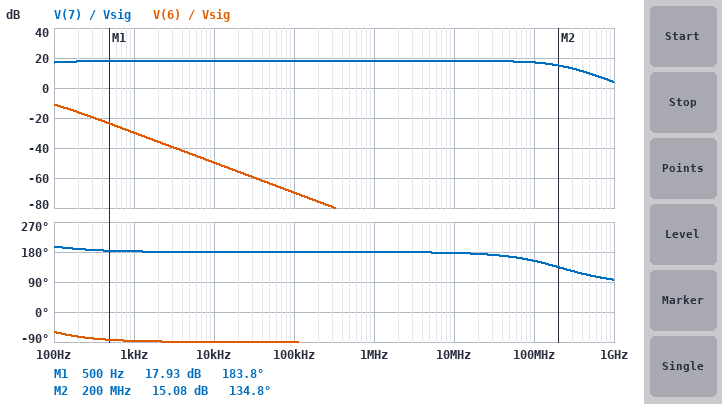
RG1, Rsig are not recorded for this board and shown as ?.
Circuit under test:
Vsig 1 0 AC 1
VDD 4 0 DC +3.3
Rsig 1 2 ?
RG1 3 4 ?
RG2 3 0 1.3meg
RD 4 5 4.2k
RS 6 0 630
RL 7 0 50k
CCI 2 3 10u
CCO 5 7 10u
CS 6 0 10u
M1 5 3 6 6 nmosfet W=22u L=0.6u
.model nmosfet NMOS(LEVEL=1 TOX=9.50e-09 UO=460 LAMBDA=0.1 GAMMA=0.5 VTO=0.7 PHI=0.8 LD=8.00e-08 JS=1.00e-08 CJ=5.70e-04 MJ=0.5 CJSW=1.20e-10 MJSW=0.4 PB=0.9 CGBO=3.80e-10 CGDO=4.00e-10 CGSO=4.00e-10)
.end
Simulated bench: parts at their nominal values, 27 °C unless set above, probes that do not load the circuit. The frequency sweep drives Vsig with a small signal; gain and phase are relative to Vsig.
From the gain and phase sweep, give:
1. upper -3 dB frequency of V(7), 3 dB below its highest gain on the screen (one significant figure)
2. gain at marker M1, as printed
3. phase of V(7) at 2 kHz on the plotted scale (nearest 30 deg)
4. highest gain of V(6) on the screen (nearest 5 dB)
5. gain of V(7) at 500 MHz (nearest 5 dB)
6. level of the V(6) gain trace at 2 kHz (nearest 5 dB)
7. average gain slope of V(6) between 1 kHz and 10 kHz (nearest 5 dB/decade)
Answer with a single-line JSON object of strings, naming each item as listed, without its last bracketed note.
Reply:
{"upper -3 dB frequency of V(7), 3 dB below its highest gain on the screen": "200 MHz", "gain at marker M1, as printed": "17.93 dB", "phase of V(7) at 2 kHz on the plotted scale": "180 deg", "highest gain of V(6) on the screen": "-10 dB", "gain of V(7) at 500 MHz": "10 dB", "level of the V(6) gain trace at 2 kHz": "-35 dB", "average gain slope of V(6) between 1 kHz and 10 kHz": "-20 dB/decade"}
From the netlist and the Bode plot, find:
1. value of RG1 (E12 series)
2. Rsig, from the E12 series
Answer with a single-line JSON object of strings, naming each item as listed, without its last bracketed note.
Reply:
{"value of RG1": "2.7 MΩ", "Rsig, from the E12 series": "6.8 kΩ"}
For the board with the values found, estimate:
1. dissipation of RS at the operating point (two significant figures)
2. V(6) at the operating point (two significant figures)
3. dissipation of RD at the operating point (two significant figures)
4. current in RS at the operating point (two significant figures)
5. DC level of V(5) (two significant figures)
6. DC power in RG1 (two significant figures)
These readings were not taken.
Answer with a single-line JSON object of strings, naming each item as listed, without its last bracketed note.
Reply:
{"dissipation of RS at the operating point": "37 µW", "V(6) at the operating point": "150 mV", "dissipation of RD at the operating point": "250 µW", "current in RS at the operating point": "240 µA", "DC level of V(5)": "2.3 V", "DC power in RG1": "1.8 µW"}
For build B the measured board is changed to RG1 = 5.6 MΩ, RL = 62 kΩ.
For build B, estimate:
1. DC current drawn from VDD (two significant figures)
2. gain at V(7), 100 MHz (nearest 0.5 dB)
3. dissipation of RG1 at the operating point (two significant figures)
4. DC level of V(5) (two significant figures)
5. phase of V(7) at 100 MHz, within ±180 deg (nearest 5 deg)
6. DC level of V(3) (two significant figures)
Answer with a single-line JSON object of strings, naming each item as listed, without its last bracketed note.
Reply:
{"DC current drawn from VDD": "480 nA", "gain at V(7), 100 MHz": "-33.5 dB", "dissipation of RG1 at the operating point": "1.3 µW", "DC level of V(5)": "3.3 V", "phase of V(7) at 100 MHz, within ±180 deg": "80 deg", "DC level of V(3)": "620 mV"}
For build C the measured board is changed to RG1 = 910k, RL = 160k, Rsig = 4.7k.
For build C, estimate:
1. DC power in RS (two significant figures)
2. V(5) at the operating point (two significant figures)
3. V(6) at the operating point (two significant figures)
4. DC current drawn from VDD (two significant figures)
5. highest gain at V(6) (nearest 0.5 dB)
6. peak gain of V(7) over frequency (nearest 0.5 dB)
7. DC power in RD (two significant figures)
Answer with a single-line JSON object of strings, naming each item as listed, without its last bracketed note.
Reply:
{"DC power in RS": "280 µW", "V(5) at the operating point": "520 mV", "V(6) at the operating point": "420 mV", "DC current drawn from VDD": "660 µA", "highest gain at V(6)": "-35.0 dB", "peak gain of V(7) over frequency": "-17.5 dB", "DC power in RD": "1.8 mW"}
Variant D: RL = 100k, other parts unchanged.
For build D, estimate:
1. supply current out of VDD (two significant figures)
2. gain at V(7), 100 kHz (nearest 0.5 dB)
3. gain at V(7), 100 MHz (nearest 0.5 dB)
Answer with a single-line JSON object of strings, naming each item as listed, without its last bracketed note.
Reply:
{"supply current out of VDD": "240 µA", "gain at V(7), 100 kHz": "18.5 dB", "gain at V(7), 100 MHz": "17.5 dB"}
